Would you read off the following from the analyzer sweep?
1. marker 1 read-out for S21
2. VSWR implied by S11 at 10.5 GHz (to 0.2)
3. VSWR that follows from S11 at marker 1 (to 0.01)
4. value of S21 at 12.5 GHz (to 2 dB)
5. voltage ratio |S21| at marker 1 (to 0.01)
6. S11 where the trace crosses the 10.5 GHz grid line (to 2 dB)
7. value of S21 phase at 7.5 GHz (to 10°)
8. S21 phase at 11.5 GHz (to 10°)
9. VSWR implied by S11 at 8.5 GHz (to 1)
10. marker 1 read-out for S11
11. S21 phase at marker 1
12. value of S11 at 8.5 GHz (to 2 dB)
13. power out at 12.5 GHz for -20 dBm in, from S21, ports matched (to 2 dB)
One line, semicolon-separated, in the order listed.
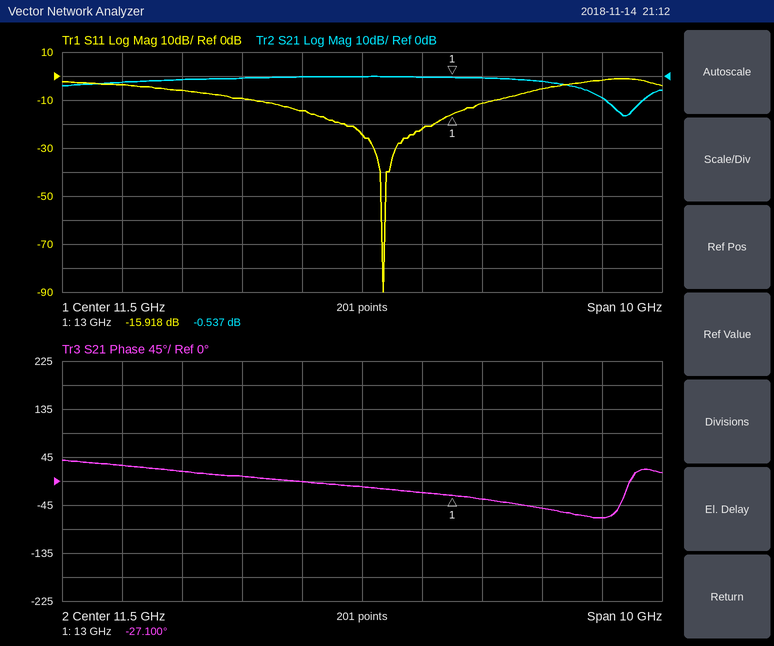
-0.537 dB; 1.4; 1.38; 0 dB; 0.94; -14 dB; 30°; -10°; 3; -15.918 dB; -27.100°; -6 dB; -20 dBm
